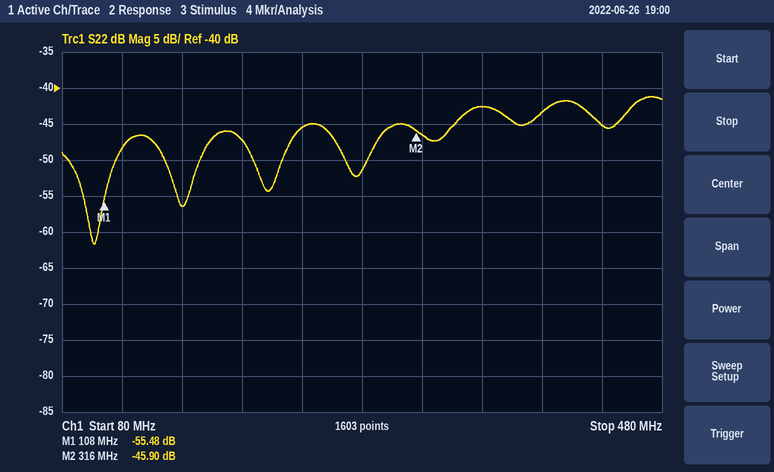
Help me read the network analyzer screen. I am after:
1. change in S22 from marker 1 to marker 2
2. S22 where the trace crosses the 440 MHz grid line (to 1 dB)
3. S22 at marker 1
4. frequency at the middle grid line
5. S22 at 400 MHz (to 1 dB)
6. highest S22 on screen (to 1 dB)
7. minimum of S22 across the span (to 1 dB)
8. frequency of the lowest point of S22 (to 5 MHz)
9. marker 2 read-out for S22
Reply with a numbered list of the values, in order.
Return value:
1. 9.58 dB
2. -45 dB
3. -55.48 dB
4. 280 MHz
5. -43 dB
6. -41 dB
7. -62 dB
8. 100 MHz
9. -45.90 dB
